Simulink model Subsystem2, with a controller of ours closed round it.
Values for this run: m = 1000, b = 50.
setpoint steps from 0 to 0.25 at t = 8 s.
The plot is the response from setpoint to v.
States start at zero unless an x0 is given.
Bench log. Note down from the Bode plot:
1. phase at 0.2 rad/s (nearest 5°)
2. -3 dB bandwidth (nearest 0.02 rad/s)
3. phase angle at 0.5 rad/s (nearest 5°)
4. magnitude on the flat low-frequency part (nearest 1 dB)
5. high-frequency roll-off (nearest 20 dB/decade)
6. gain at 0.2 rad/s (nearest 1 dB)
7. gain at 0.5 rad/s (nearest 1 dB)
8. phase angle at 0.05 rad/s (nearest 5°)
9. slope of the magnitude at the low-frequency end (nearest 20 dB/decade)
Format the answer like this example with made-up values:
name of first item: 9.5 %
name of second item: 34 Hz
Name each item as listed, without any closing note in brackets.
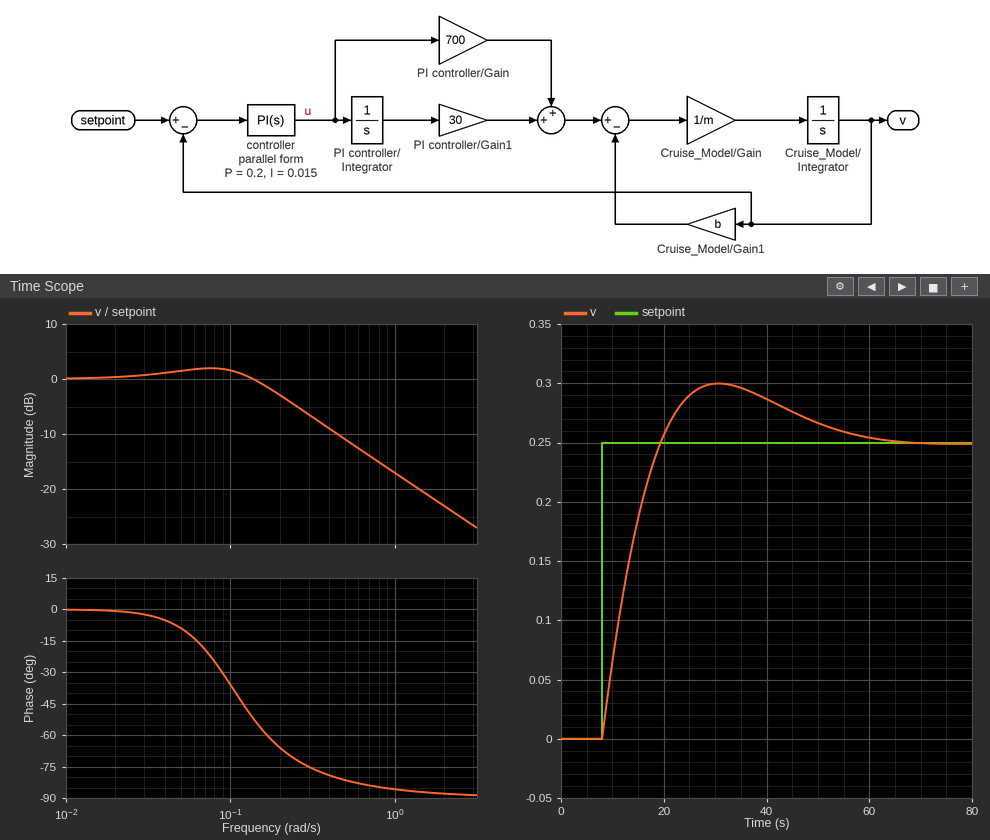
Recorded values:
phase at 0.2 rad/s: -65°
-3 dB bandwidth: 0.20 rad/s
phase angle at 0.5 rad/s: -80°
magnitude on the flat low-frequency part: 0 dB
high-frequency roll-off: -20 dB/decade
gain at 0.2 rad/s: -3 dB
gain at 0.5 rad/s: -11 dB
phase angle at 0.05 rad/s: -10°
slope of the magnitude at the low-frequency end: 0 dB/decade
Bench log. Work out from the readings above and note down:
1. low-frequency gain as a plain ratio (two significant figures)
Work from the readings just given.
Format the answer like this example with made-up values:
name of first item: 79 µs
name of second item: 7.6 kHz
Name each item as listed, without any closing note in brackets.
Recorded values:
low-frequency gain as a plain ratio: 1.0
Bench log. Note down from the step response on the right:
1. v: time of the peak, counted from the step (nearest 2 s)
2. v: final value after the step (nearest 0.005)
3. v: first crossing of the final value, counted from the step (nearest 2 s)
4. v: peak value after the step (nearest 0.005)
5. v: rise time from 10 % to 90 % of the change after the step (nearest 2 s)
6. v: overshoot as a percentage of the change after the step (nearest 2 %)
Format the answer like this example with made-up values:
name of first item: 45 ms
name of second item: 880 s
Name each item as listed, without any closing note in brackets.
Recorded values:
v: time of the peak, counted from the step: 22 s
v: final value after the step: 0.250
v: first crossing of the final value, counted from the step: 12 s
v: peak value after the step: 0.300
v: rise time from 10 % to 90 % of the change after the step: 8 s
v: overshoot as a percentage of the change after the step: 20 %
